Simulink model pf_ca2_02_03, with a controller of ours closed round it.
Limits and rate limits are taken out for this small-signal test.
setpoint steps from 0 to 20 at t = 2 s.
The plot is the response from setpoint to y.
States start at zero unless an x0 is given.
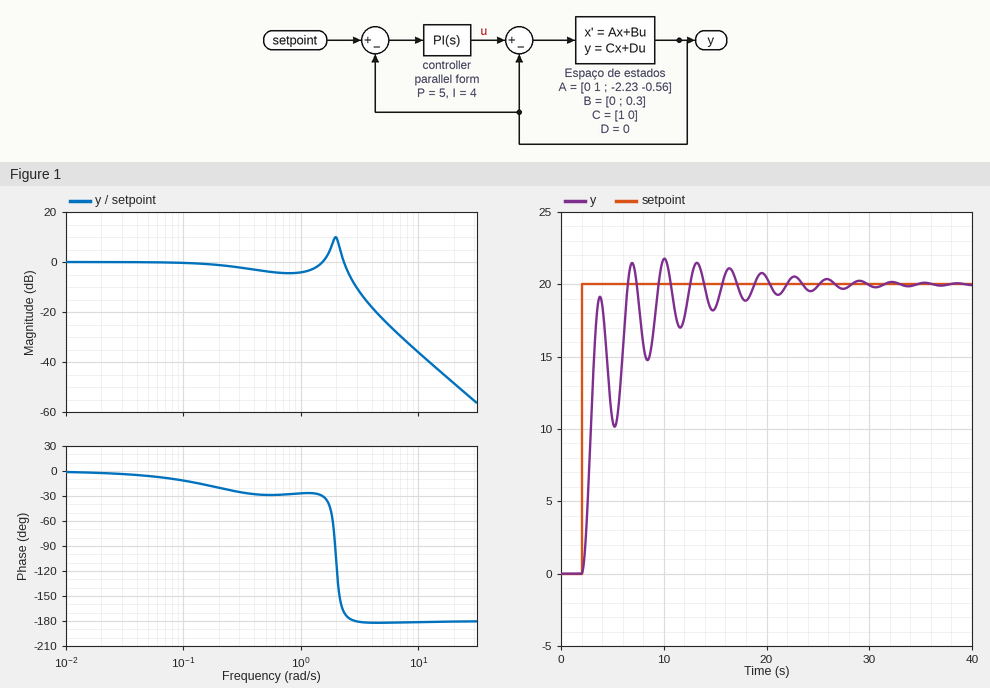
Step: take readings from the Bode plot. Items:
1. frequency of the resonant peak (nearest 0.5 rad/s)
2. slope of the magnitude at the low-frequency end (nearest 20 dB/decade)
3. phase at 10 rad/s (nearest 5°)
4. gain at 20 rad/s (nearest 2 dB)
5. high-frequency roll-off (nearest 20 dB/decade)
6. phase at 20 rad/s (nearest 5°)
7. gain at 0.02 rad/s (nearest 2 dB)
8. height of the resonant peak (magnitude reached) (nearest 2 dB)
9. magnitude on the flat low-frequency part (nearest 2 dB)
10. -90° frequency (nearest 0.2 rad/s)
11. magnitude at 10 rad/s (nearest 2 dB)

2.0 rad/s
0 dB/decade
-180°
-48 dB
-40 dB/decade
-180°
0 dB
10 dB
0 dB
2.0 rad/s
-36 dB
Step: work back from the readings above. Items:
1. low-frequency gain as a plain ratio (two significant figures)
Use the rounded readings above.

1.0
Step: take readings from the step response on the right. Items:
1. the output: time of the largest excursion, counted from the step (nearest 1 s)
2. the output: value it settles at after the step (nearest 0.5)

8 s
20.0
